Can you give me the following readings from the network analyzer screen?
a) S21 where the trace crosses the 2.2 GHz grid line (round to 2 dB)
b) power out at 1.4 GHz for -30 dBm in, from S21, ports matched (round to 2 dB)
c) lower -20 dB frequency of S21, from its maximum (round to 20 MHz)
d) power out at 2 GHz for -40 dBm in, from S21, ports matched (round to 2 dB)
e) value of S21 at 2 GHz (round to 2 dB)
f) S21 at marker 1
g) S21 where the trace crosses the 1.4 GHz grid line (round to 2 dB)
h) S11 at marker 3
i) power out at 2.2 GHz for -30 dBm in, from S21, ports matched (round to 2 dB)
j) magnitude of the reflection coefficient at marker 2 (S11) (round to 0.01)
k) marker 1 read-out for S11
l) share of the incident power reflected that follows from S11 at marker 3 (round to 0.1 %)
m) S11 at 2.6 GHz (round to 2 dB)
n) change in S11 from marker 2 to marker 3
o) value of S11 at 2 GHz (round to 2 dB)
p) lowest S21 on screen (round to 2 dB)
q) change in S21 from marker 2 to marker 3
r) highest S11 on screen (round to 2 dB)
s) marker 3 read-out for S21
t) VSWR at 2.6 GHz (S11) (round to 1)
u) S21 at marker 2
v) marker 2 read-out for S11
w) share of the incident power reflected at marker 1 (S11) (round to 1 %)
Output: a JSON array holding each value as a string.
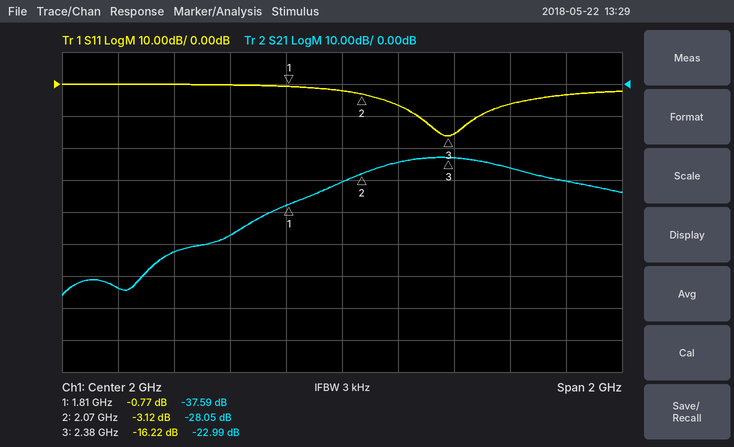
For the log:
["-24 dB", "-82 dBm", "1.68 GHz", "-70 dBm", "-30 dB", "-37.59 dB", "-52 dB", "-16.22 dB", "-54 dBm", "0.70", "-0.77 dB", "2.4 %", "-6 dB", "-13.10 dB", "-2 dB", "-66 dB", "5.06 dB", "0 dB", "-22.99 dB", "3", "-28.05 dB", "-3.12 dB", "84 %"]
